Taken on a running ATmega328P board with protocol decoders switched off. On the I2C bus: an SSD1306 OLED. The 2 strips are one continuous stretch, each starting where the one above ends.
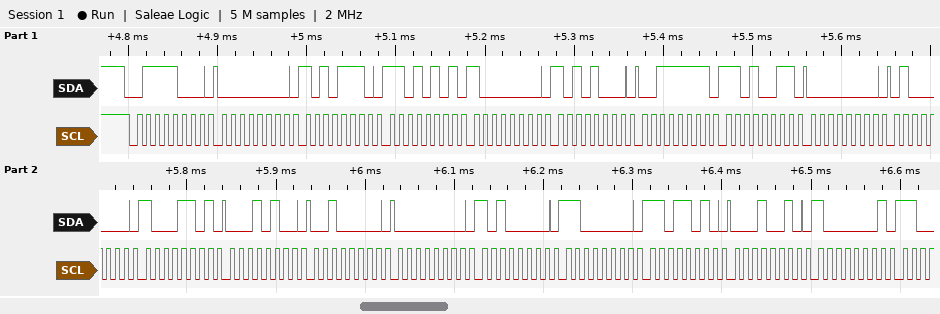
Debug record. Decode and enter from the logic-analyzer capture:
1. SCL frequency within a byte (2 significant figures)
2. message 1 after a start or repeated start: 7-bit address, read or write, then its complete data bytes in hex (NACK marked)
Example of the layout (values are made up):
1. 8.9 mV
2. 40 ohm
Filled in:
1. 100 kHz
2. 0x3C write: 00 AE D5 80 A8 3F D3 00 40 8D 14 20 00 A0 C0 DA 12 81
